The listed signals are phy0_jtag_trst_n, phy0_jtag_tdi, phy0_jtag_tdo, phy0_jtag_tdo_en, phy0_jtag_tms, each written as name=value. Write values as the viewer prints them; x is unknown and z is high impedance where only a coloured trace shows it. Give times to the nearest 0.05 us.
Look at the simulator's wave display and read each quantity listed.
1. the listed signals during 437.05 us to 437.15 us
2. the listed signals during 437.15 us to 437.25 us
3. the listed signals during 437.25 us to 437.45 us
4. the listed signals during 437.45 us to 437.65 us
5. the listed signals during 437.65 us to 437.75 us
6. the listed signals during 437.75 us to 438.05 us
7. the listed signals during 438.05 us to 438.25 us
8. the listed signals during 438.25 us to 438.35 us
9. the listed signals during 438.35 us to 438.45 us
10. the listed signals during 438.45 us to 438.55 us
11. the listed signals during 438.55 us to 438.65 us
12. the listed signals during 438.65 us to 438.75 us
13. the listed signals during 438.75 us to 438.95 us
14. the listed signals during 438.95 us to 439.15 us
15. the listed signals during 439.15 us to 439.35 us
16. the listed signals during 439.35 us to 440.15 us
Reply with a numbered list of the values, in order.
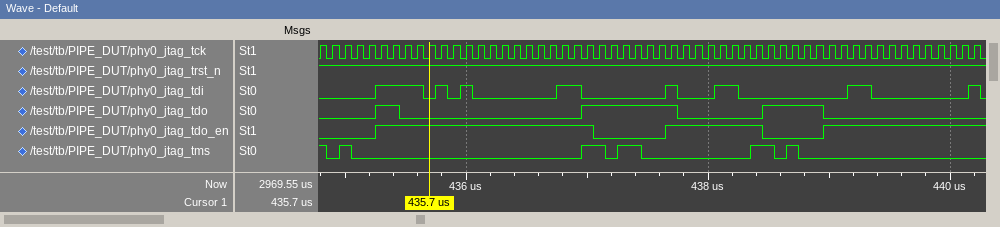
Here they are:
1. phy0_jtag_trst_n=1, phy0_jtag_tdi=0, phy0_jtag_tdo=1, phy0_jtag_tdo_en=0, phy0_jtag_tms=1
2. phy0_jtag_trst_n=1, phy0_jtag_tdi=0, phy0_jtag_tdo=1, phy0_jtag_tdo_en=0, phy0_jtag_tms=0
3. phy0_jtag_trst_n=1, phy0_jtag_tdi=0, phy0_jtag_tdo=1, phy0_jtag_tdo_en=0, phy0_jtag_tms=1
4. phy0_jtag_trst_n=1, phy0_jtag_tdi=0, phy0_jtag_tdo=1, phy0_jtag_tdo_en=0, phy0_jtag_tms=0
5. phy0_jtag_trst_n=1, phy0_jtag_tdi=1, phy0_jtag_tdo=1, phy0_jtag_tdo_en=1, phy0_jtag_tms=0
6. phy0_jtag_trst_n=1, phy0_jtag_tdi=0, phy0_jtag_tdo=0, phy0_jtag_tdo_en=1, phy0_jtag_tms=0
7. phy0_jtag_trst_n=1, phy0_jtag_tdi=1, phy0_jtag_tdo=0, phy0_jtag_tdo_en=1, phy0_jtag_tms=0
8. phy0_jtag_trst_n=1, phy0_jtag_tdi=0, phy0_jtag_tdo=0, phy0_jtag_tdo_en=1, phy0_jtag_tms=0
9. phy0_jtag_trst_n=1, phy0_jtag_tdi=0, phy0_jtag_tdo=0, phy0_jtag_tdo_en=1, phy0_jtag_tms=1
10. phy0_jtag_trst_n=1, phy0_jtag_tdi=0, phy0_jtag_tdo=1, phy0_jtag_tdo_en=0, phy0_jtag_tms=1
11. phy0_jtag_trst_n=1, phy0_jtag_tdi=0, phy0_jtag_tdo=1, phy0_jtag_tdo_en=0, phy0_jtag_tms=0
12. phy0_jtag_trst_n=1, phy0_jtag_tdi=0, phy0_jtag_tdo=1, phy0_jtag_tdo_en=0, phy0_jtag_tms=1
13. phy0_jtag_trst_n=1, phy0_jtag_tdi=0, phy0_jtag_tdo=1, phy0_jtag_tdo_en=0, phy0_jtag_tms=0
14. phy0_jtag_trst_n=1, phy0_jtag_tdi=0, phy0_jtag_tdo=0, phy0_jtag_tdo_en=1, phy0_jtag_tms=0
15. phy0_jtag_trst_n=1, phy0_jtag_tdi=1, phy0_jtag_tdo=0, phy0_jtag_tdo_en=1, phy0_jtag_tms=0
16. phy0_jtag_trst_n=1, phy0_jtag_tdi=0, phy0_jtag_tdo=0, phy0_jtag_tdo_en=1, phy0_jtag_tms=0
